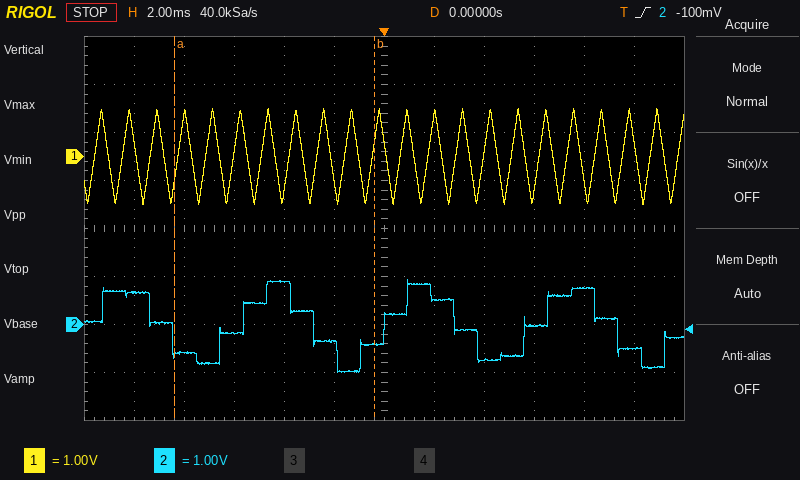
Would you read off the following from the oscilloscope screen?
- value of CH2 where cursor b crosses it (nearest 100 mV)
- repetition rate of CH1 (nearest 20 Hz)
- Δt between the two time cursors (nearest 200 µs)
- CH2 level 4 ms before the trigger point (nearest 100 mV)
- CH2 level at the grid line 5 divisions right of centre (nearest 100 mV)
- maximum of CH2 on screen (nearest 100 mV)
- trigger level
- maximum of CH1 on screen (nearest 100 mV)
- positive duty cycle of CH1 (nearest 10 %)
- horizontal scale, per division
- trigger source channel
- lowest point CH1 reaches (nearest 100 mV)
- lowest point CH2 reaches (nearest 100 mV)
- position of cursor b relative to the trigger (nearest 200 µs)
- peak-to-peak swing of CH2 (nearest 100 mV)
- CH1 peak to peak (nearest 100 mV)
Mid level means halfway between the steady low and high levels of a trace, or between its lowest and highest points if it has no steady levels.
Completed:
-400 mV
900 Hz
8.0 ms
900 mV
-500 mV
900 mV
-100 mV
1.0 V
50 %
2 ms
CH2
-1.0 V
-1.0 V
-400 µs
1.9 V
2.0 V
